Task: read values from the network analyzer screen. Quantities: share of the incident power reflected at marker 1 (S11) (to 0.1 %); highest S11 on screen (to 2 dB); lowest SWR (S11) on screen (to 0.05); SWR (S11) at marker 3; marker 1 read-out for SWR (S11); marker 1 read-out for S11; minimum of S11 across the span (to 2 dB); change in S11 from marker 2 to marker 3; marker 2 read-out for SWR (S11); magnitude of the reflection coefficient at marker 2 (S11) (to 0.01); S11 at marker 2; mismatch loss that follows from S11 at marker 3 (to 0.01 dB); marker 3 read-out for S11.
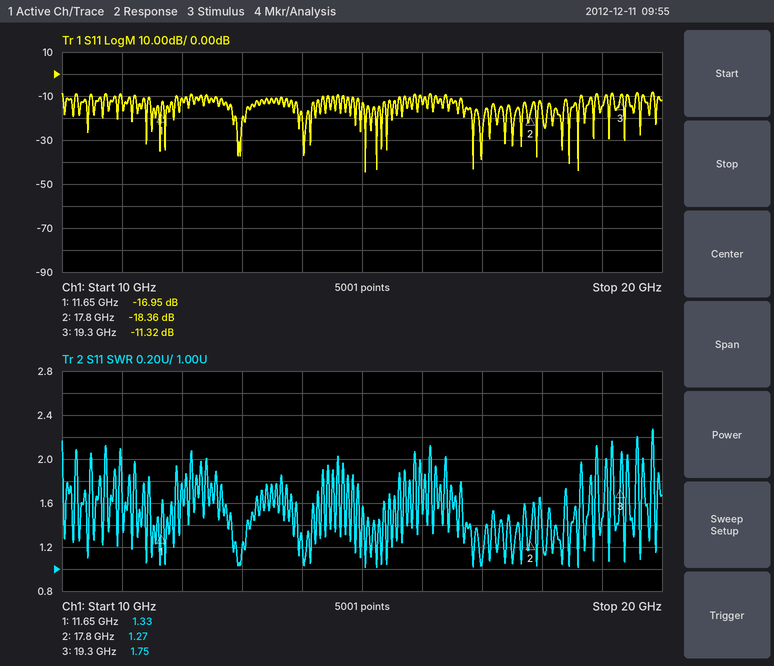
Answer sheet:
2.0 %
-8 dB
1.00
1.75
1.33
-16.95 dB
-44 dB
7.04 dB
1.27
0.12
-18.36 dB
0.33 dB
-11.32 dB
